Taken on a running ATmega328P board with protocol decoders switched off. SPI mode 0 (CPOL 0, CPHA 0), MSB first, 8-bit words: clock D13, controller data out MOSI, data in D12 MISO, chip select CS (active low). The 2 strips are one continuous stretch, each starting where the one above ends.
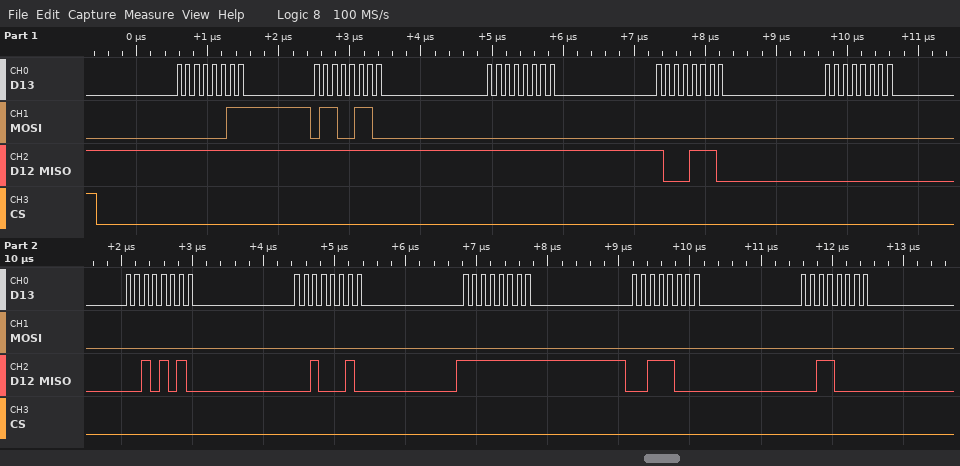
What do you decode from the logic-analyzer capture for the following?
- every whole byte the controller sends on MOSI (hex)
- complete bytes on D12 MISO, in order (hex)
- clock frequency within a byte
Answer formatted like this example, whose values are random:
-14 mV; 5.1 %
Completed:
0x03 0x66 0x00 0x00 0x00 0x00 0x00 0x00 0x00 0x00; 0xFF 0xFF 0xFF 0x8E 0x00 0x2A 0x22 0xFF 0x38 0x30; 8 MHz
